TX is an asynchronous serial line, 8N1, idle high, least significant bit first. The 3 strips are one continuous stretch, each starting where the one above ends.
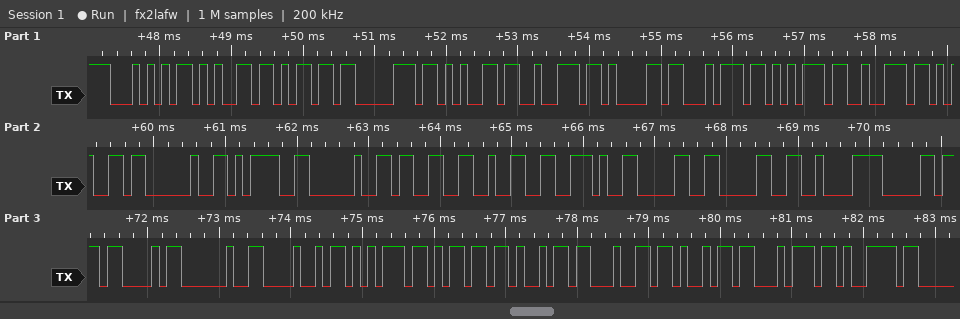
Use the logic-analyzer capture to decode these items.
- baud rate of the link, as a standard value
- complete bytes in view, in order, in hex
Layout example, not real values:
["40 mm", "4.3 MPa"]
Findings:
["9600 baud", "0x54 0x65 0x6D 0x70 0x65 0x72 0x61 0x74 0x75 0x72 0x65 0x20 0x3D 0x20 0x33 0x32 0x2E 0x30 0x30 0xC2 0xB0 0x43 0x20 0x48 0x75 0x6D 0x69 0x64 0x69 0x74 0x79"]
